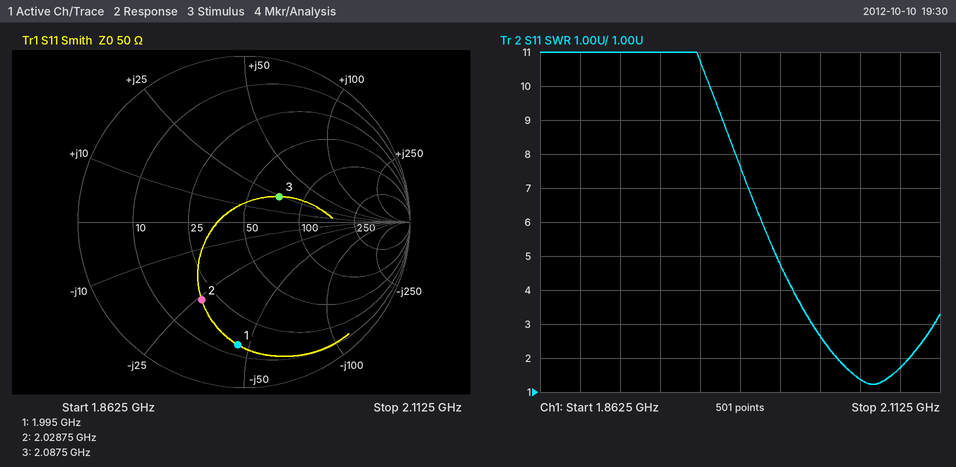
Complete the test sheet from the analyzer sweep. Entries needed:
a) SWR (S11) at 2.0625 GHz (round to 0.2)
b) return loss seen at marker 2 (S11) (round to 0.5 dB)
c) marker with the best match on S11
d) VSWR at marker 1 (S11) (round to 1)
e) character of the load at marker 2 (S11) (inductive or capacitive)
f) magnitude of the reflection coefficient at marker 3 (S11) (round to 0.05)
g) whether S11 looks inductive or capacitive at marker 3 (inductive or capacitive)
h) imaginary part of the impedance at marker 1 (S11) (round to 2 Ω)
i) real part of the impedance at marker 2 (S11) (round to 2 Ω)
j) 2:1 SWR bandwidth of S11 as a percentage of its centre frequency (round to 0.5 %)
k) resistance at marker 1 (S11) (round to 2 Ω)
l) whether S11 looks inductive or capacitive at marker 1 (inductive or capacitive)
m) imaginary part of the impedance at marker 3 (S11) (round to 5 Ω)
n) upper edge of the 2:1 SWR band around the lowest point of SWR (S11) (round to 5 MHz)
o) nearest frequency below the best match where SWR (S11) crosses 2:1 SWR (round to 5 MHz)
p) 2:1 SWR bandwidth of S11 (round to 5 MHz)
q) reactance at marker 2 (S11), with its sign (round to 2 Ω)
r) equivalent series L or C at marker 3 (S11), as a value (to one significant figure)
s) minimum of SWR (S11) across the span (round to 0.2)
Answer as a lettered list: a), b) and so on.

a) 1.4
b) 5.5 dB
c) marker 3
d) 7
e) capacitive
f) 0.25
g) inductive
h) -46 Ω
i) 20 Ω
j) 2.0 %
k) 14 Ω
l) capacitive
m) +25 Ω
n) 2.095 GHz
o) 2.050 GHz
p) 45 MHz
q) -26 Ω
r) 2 nH
s) 1.2
